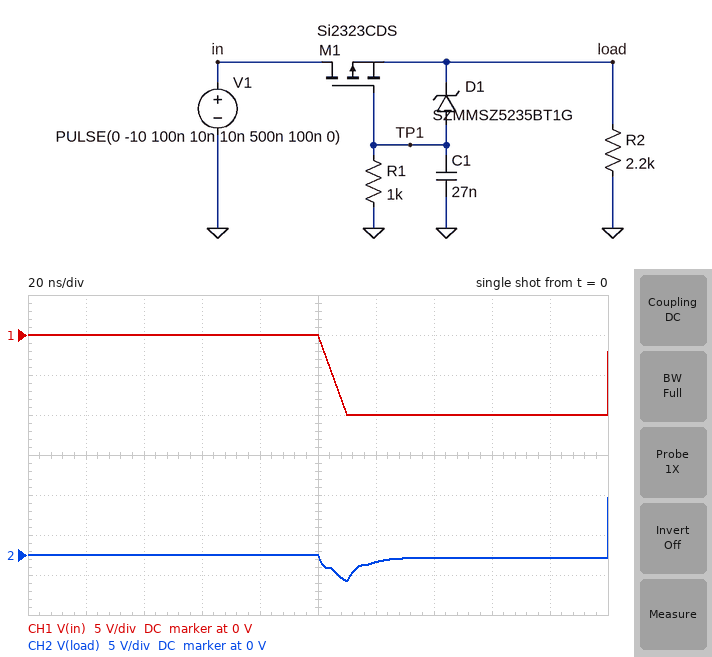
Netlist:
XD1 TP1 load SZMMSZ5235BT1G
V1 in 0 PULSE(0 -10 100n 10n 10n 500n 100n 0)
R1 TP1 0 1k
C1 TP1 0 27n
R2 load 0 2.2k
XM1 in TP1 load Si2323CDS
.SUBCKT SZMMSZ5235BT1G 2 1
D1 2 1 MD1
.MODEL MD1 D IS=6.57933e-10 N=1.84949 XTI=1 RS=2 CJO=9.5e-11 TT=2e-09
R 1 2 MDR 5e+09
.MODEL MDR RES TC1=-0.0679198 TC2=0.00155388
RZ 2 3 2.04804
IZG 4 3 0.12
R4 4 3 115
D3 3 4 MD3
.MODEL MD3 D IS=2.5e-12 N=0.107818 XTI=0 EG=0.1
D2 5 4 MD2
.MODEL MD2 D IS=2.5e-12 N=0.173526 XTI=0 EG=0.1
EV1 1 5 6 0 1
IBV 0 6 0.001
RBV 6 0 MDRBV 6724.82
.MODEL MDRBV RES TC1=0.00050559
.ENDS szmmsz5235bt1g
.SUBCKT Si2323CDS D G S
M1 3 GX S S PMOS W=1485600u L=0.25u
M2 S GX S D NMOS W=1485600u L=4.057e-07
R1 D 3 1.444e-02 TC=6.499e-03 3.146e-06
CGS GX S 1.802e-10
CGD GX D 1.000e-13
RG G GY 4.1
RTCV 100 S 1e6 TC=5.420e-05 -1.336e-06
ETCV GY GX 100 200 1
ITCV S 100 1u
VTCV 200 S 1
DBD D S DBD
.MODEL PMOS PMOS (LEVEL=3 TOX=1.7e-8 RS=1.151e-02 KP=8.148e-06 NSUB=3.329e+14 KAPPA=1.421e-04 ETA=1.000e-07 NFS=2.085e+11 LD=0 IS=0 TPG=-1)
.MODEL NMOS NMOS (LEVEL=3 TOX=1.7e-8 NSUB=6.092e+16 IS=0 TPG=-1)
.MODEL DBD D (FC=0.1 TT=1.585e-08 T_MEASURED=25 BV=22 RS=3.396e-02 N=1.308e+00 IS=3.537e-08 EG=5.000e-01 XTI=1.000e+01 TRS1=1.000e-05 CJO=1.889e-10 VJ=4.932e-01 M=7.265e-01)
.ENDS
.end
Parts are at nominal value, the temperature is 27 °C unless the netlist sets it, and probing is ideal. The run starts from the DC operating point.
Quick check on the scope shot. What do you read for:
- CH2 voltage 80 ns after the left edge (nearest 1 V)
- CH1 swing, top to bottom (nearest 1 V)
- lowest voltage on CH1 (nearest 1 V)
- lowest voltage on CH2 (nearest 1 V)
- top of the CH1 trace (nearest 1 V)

0 V
10 V
-10 V
-3 V
0 V
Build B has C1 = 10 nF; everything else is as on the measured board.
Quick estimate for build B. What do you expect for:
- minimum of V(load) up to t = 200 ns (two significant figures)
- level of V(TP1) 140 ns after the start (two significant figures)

-3.6 V
-1.5 V
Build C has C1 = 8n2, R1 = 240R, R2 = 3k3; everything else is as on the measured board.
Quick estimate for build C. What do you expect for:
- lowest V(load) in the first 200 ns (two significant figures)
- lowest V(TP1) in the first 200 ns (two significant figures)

-3.7 V
-1.7 V
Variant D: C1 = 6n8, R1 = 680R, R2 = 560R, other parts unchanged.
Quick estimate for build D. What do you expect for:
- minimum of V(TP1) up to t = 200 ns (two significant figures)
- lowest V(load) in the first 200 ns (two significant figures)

-2.0 V
-3.8 V
